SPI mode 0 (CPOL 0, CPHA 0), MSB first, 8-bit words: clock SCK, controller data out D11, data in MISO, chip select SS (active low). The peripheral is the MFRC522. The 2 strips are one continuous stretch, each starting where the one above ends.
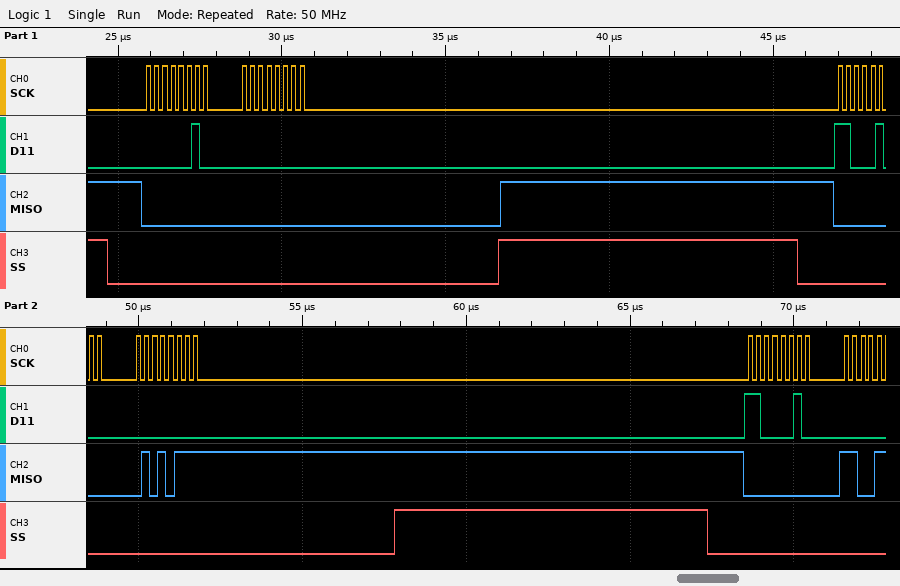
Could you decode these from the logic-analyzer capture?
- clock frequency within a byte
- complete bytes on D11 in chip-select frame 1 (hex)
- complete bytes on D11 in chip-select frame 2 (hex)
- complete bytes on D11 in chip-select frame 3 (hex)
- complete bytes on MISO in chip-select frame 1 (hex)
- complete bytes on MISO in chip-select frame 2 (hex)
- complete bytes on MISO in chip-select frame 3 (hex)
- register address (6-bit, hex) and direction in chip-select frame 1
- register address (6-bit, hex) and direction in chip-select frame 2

4 MHz
0x02 0x00
0xC4 0x00
0xC2
0x00 0x00
0x00 0x57
0x00
0x01 write
0x22 read
